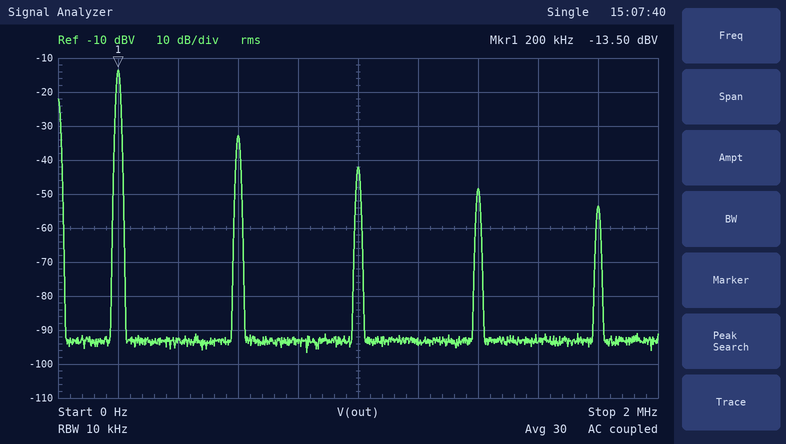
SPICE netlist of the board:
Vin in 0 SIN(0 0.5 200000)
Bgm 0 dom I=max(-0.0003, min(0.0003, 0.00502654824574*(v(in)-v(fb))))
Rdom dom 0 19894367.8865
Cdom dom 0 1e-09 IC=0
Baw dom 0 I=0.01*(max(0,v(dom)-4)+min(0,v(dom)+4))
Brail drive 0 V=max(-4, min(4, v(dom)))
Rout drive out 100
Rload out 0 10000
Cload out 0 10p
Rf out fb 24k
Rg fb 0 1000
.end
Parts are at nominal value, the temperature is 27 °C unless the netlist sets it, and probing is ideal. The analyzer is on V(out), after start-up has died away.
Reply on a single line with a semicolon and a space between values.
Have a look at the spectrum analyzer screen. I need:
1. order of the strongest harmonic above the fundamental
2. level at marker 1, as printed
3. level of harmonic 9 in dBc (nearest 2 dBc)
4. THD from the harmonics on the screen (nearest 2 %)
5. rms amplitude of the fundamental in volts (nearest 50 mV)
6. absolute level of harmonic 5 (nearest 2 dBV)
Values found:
3; -13.50 dBV; -40 dBc; 12 %; 200 mV; -42 dBV
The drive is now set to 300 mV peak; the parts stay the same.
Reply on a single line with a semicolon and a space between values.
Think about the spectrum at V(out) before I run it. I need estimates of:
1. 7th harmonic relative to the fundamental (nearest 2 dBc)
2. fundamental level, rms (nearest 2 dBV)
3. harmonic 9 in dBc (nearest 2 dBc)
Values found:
-36 dBc; -14 dBV; -44 dBc
